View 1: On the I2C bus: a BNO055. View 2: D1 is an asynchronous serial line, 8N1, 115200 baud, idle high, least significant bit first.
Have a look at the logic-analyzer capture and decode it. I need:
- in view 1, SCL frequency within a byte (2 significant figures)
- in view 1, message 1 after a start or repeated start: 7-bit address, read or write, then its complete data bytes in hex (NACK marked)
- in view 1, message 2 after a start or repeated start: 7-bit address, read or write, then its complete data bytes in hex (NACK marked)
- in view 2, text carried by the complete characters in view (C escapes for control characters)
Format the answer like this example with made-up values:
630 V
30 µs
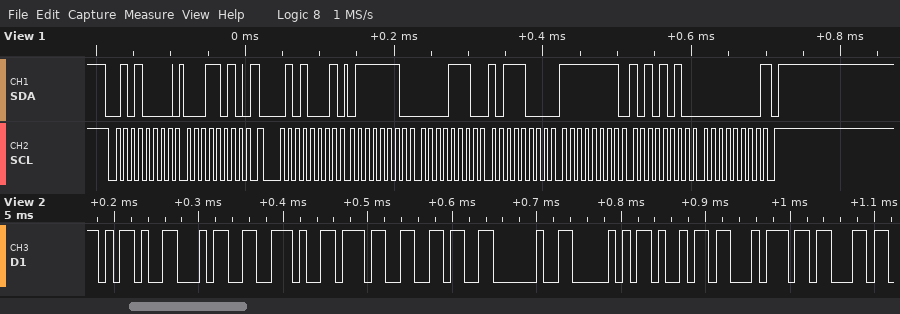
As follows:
100 kHz
0x28 write: 1A
0x28 read: 7E 0E B8 FF AA 00 NACK
"-4.76 Pitc"
